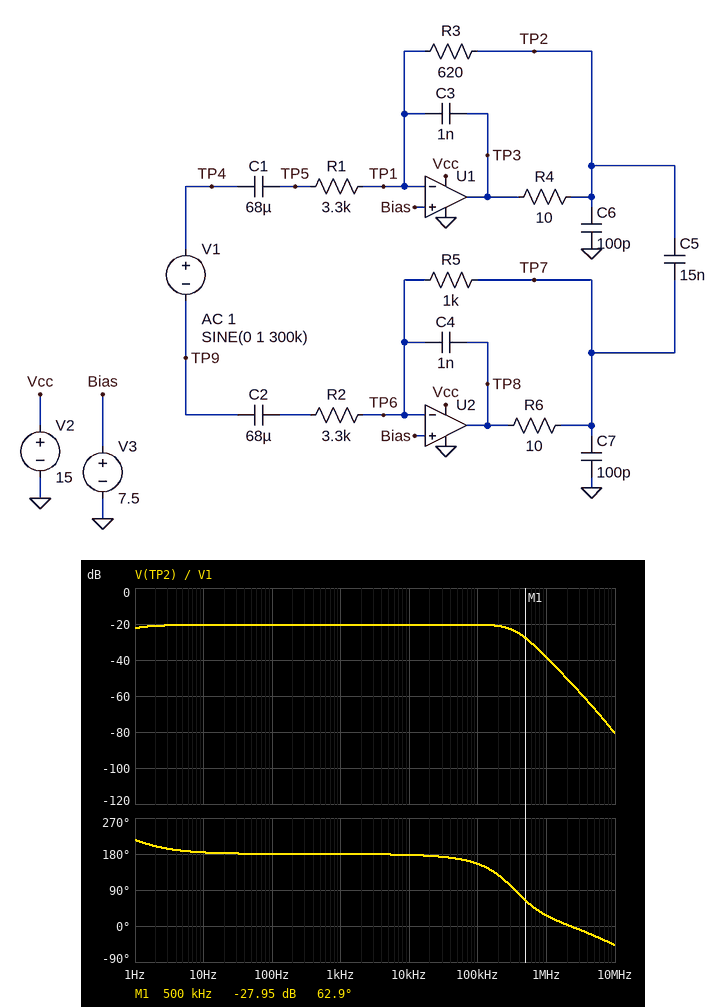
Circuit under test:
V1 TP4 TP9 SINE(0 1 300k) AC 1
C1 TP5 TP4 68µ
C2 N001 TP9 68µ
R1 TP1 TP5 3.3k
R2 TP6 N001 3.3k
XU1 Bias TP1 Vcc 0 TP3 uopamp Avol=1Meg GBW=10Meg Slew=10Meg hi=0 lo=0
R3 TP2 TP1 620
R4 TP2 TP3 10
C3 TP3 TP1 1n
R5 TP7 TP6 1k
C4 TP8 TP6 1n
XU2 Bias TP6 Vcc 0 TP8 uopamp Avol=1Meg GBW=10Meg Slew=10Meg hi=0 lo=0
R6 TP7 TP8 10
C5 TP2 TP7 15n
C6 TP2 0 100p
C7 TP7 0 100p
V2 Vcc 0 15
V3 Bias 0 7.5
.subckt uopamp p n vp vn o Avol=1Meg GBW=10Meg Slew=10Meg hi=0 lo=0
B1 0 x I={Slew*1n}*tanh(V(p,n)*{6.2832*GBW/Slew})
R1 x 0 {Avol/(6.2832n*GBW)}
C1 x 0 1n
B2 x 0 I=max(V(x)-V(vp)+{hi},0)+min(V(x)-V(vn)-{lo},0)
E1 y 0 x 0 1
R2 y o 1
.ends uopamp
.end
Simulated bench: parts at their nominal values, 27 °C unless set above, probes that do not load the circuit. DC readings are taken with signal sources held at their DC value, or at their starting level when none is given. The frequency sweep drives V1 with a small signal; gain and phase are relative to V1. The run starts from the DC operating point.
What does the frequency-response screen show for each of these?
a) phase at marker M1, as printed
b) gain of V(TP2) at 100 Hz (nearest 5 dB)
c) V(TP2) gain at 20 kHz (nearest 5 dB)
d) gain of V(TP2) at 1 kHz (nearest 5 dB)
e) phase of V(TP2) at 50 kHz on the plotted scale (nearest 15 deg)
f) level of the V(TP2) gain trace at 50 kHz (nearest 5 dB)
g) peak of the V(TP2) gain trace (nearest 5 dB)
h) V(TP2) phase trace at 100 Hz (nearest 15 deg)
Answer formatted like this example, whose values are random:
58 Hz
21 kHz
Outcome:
62.9 deg
-20 dB
-20 dB
-20 dB
165 deg
-20 dB
-20 dB
180 deg
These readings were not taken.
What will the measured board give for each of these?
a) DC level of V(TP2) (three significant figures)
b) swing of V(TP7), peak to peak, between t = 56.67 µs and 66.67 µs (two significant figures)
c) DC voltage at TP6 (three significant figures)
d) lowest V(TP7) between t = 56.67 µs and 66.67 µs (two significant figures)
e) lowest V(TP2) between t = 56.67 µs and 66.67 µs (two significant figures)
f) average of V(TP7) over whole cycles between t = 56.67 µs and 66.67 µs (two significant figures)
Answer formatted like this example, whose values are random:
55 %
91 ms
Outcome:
7.50 V
170 mV
7.50 V
7.4 V
7.4 V
7.5 V
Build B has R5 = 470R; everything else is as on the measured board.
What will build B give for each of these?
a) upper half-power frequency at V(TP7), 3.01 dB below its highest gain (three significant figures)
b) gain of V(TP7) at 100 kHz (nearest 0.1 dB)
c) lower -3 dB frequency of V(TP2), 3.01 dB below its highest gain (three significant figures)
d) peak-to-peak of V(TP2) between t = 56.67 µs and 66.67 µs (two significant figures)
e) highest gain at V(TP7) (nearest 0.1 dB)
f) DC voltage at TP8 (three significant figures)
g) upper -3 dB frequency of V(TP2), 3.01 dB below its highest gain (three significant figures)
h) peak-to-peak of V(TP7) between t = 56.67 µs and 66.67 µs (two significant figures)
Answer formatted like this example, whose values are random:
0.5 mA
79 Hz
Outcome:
428 kHz
-22.8 dB
709 mHz
160 mV
-22.7 dB
7.50 V
371 kHz
140 mV
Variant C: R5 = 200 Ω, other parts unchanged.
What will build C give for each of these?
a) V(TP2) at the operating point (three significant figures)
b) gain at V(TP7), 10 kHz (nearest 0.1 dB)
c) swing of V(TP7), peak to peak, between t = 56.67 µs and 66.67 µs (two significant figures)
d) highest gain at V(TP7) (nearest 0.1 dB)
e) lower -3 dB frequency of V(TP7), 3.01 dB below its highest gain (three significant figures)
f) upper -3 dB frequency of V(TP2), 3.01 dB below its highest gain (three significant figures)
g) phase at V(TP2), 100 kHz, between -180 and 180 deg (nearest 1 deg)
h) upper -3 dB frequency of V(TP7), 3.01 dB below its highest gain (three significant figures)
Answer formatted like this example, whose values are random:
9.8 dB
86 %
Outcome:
7.50 V
-30.4 dB
72 mV
-28.8 dB
1.13 Hz
393 kHz
157 deg
631 kHz
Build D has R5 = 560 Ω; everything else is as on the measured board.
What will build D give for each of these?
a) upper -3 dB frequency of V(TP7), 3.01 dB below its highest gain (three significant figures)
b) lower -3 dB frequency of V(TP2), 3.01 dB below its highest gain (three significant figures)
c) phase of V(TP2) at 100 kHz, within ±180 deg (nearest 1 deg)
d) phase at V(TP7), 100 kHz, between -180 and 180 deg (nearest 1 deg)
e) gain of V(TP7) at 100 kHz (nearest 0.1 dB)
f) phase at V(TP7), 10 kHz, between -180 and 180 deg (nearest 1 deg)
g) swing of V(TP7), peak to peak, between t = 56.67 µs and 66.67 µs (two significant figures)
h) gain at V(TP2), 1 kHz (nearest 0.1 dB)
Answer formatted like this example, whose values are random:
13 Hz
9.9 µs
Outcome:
385 kHz
709 mHz
156 deg
-22 deg
-21.4 dB
-2 deg
150 mV
-20.5 dB
